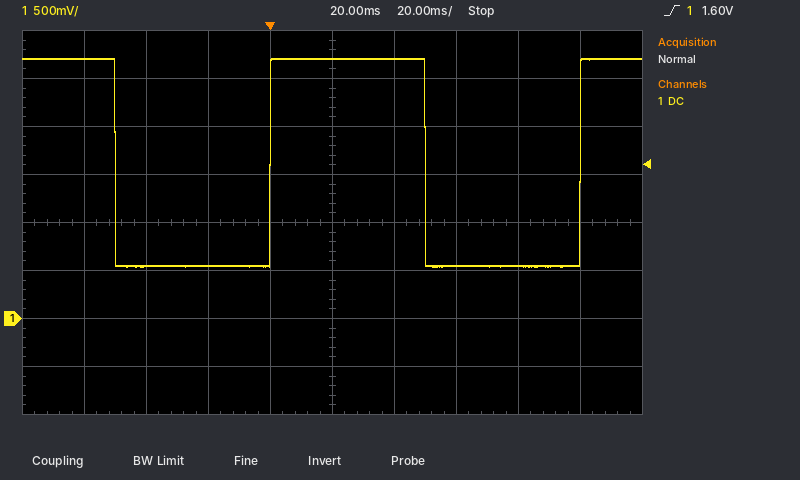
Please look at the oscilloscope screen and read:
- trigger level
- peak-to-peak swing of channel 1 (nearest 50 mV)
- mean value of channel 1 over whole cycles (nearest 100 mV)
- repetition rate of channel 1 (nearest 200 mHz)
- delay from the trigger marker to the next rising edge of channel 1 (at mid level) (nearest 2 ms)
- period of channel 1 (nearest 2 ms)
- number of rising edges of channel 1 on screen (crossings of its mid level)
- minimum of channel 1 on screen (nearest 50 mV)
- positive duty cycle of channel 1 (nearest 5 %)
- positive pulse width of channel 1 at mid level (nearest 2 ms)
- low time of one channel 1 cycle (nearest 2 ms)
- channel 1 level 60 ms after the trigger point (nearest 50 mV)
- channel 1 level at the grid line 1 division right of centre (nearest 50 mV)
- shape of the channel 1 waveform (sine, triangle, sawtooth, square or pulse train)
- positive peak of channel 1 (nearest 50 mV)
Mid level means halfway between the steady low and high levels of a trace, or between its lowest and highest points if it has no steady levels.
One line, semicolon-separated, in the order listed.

1.60 V; 2.15 V; 1.6 V; 10.0 Hz; 100 ms; 100 ms; 2; 550 mV; 50 %; 50 ms; 50 ms; 550 mV; 2.70 V; square; 2.70 V
